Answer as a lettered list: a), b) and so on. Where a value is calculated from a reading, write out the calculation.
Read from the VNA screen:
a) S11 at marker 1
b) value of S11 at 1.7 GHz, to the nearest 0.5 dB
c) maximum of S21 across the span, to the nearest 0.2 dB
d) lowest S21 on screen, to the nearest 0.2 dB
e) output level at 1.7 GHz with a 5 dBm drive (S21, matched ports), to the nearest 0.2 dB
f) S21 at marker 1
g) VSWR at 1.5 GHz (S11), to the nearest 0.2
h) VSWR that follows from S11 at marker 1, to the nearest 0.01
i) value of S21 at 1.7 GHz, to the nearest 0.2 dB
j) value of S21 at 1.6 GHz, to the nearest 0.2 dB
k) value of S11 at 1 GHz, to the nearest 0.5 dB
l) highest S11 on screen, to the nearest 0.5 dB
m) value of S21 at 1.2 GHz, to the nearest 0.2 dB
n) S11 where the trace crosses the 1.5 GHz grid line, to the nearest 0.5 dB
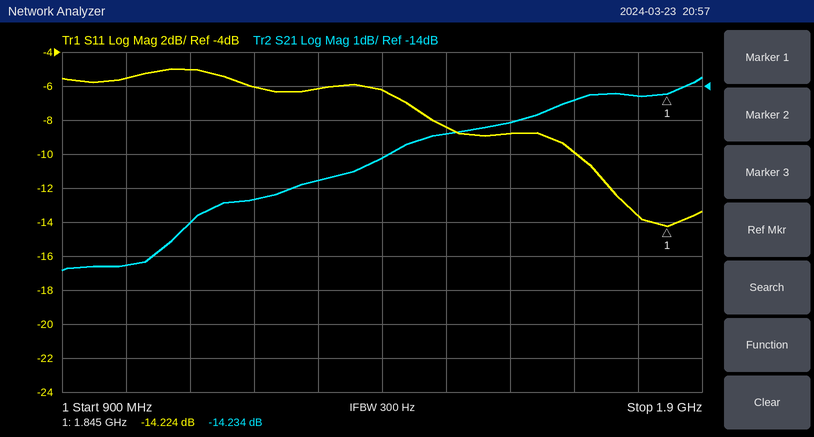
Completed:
a) -14.224 dB
b) -10.0 dB
c) -13.8 dB
d) -19.4 dB
e) 5 dBm + (-14.4 dB) = -9.4 dBm
f) -14.234 dB
g) |Γ| = 10^(-8.5/20) = 0.3758; VSWR = (1 + 0.3758)/(1 − 0.3758) ≈ 2.2
h) (1 + 0.1944)/(1 − 0.1944) ≈ 1.48
i) -14.4 dB
j) -15.0 dB
k) -5.5 dB
l) -5.0 dB
m) -17.4 dB
n) -8.5 dB
